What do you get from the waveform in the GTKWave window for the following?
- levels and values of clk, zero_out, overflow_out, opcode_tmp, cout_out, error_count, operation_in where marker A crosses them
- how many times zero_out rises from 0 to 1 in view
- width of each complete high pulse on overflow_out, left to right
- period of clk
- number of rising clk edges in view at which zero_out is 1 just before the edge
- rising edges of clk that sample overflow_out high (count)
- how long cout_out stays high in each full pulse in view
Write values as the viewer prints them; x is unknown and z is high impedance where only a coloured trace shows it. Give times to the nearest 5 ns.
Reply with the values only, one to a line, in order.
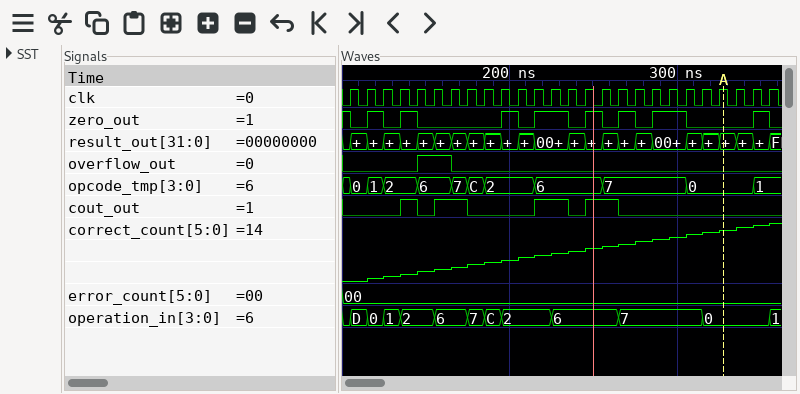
clk=1, zero_out=0, overflow_out=0, opcode_tmp=0, cout_out=0, error_count=00, operation_in=0
8
20 ns
10 ns
11
2
10 ns, 20 ns, 20 ns, 20 ns
